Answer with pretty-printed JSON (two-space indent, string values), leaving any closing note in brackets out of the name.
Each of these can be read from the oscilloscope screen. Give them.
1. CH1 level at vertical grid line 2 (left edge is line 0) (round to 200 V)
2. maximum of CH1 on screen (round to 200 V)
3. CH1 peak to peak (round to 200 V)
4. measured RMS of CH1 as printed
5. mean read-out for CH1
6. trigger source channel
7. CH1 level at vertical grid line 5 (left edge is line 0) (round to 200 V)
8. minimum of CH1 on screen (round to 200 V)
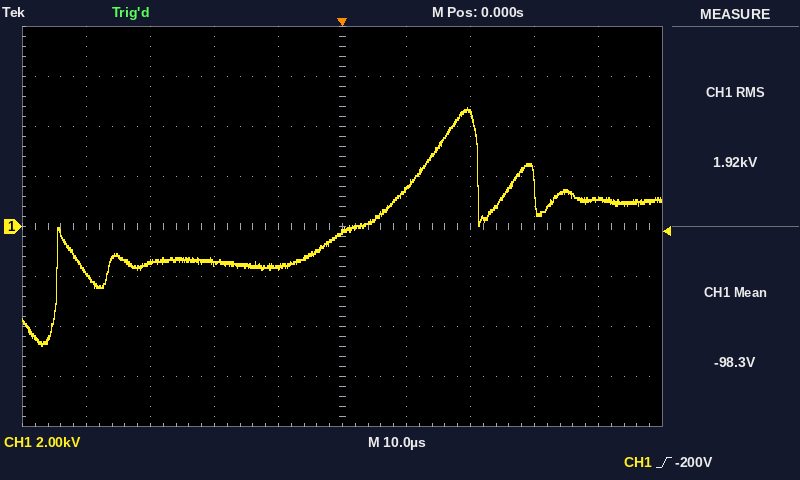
{
  "CH1 level at vertical grid line 2 (left edge is line 0)": "-1.4 kV",
  "maximum of CH1 on screen": "4.8 kV",
  "CH1 peak to peak": "9.6 kV",
  "measured RMS of CH1 as printed": "1.92 kV",
  "mean read-out for CH1": "-98.3 V",
  "trigger source channel": "CH1",
  "CH1 level at vertical grid line 5 (left edge is line 0)": "-200 V",
  "minimum of CH1 on screen": "-4.8 kV"
}
